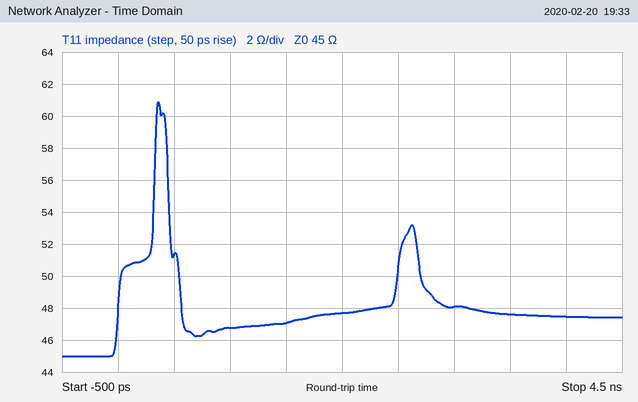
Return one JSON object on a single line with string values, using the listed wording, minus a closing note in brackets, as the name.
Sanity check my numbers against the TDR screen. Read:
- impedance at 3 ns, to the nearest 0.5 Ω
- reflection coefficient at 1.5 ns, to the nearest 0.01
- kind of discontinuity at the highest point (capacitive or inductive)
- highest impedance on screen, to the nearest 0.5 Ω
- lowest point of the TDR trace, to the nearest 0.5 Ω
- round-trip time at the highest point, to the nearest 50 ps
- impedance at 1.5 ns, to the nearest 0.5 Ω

{"impedance at 3 ns, to the nearest 0.5 Ω": "48.0 Ω", "reflection coefficient at 1.5 ns, to the nearest 0.01": "+0.02", "kind of discontinuity at the highest point": "inductive", "highest impedance on screen, to the nearest 0.5 Ω": "61.0 Ω", "lowest point of the TDR trace, to the nearest 0.5 Ω": "45.0 Ω", "round-trip time at the highest point, to the nearest 50 ps": "350 ps", "impedance at 1.5 ns, to the nearest 0.5 Ω": "47.0 Ω"}
